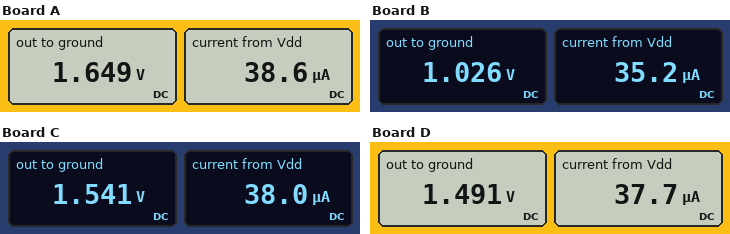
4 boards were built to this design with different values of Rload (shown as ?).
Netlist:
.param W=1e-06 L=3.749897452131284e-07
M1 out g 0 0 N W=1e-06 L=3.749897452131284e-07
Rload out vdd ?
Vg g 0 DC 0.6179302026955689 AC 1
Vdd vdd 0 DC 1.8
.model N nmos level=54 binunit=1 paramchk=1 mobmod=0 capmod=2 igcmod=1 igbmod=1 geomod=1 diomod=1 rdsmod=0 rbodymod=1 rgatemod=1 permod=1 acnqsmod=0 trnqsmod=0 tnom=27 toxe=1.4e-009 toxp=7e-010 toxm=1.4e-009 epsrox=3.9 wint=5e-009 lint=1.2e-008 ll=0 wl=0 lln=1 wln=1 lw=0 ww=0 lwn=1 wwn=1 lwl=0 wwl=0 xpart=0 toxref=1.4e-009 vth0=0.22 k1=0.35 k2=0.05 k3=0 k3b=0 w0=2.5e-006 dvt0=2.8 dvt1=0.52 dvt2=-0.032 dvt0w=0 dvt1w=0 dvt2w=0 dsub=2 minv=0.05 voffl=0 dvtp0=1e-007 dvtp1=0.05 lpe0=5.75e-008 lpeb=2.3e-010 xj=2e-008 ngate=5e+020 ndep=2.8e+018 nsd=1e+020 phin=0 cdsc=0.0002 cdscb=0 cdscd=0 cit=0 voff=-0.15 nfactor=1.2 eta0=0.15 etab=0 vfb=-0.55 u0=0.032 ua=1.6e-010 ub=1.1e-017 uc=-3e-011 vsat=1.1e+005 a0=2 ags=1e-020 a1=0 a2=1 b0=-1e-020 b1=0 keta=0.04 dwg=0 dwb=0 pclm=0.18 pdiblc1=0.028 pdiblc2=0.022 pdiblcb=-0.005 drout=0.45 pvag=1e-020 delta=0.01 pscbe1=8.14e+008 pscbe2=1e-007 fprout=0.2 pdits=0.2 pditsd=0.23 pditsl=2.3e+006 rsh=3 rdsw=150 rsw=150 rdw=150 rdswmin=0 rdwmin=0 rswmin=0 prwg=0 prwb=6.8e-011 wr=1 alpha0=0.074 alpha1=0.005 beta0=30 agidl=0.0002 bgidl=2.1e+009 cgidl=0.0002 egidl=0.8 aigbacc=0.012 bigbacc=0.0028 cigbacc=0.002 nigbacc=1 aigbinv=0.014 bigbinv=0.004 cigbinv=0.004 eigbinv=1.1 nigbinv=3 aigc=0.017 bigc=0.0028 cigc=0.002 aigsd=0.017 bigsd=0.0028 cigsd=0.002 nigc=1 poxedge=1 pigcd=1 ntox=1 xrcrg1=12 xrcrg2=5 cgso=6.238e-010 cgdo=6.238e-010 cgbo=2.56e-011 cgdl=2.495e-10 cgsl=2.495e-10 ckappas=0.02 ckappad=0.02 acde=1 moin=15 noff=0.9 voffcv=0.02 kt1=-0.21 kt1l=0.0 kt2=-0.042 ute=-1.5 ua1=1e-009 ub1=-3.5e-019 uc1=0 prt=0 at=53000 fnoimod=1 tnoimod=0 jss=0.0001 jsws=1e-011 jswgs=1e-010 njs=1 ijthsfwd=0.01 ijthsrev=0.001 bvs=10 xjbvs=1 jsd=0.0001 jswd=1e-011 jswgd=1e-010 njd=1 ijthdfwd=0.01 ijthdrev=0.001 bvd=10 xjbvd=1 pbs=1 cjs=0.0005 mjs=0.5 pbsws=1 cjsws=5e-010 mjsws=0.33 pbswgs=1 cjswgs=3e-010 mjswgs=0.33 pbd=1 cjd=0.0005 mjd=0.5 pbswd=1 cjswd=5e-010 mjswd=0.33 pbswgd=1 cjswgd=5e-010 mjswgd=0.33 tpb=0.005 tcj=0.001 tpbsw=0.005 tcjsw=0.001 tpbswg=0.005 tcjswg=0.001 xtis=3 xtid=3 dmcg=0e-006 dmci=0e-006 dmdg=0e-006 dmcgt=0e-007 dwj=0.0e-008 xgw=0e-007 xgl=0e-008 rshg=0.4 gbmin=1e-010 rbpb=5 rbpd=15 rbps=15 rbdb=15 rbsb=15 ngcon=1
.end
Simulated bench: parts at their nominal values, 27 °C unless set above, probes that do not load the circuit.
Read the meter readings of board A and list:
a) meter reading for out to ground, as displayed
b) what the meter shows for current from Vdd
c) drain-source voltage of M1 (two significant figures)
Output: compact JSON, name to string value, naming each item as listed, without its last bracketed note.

{"meter reading for out to ground, as displayed": "1.649 V", "what the meter shows for current from Vdd": "38.6 µA", "drain-source voltage of M1": "1.6 V"}
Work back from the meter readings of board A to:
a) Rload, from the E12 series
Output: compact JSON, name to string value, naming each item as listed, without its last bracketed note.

{"Rload, from the E12 series": "3.9 kΩ"}
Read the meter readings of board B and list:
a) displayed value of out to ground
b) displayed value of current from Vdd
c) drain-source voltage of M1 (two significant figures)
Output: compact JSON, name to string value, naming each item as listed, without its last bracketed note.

{"displayed value of out to ground": "1.026 V", "displayed value of current from Vdd": "35.2 µA", "drain-source voltage of M1": "1.0 V"}
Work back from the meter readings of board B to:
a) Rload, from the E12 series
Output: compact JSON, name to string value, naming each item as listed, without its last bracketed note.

{"Rload, from the E12 series": "22 kΩ"}
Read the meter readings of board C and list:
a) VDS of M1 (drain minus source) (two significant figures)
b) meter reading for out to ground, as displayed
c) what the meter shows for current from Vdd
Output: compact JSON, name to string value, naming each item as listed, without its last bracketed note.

{"VDS of M1 (drain minus source)": "1.5 V", "meter reading for out to ground, as displayed": "1.541 V", "what the meter shows for current from Vdd": "38.0 µA"}
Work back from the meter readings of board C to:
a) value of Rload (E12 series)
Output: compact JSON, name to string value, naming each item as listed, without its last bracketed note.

{"value of Rload": "6.8 kΩ"}
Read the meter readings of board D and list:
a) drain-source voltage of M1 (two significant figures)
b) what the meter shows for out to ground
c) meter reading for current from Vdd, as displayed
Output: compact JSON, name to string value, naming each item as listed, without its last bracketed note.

{"drain-source voltage of M1": "1.5 V", "what the meter shows for out to ground": "1.491 V", "meter reading for current from Vdd, as displayed": "37.7 µA"}
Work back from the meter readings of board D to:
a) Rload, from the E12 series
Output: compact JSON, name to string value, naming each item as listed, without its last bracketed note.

{"Rload, from the E12 series": "8.2 kΩ"}
